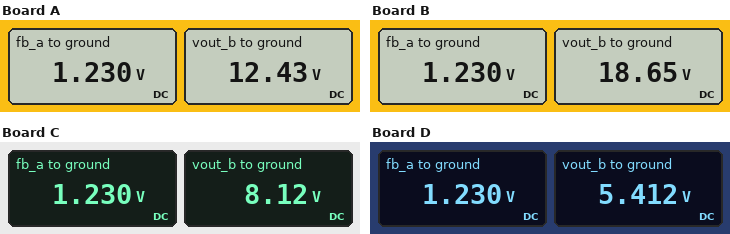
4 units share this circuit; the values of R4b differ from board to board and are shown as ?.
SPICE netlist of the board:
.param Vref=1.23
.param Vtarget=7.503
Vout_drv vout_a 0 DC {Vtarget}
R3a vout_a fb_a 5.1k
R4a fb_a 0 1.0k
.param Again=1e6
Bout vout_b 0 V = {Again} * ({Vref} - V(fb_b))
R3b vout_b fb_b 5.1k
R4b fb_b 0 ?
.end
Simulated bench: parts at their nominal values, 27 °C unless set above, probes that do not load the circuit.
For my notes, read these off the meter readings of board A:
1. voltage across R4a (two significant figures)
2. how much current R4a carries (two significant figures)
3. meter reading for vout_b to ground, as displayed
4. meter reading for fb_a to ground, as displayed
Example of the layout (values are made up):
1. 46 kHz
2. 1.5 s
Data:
1. 1.2 V
2. 1.2 mA
3. 12.43 V
4. 1.230 V
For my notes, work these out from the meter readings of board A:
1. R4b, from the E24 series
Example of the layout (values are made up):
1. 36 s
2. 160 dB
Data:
1. 560 Ω
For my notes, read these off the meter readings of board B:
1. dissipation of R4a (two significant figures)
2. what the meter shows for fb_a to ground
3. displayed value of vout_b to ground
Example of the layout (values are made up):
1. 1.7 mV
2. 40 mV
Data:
1. 1.5 mW
2. 1.230 V
3. 18.65 V
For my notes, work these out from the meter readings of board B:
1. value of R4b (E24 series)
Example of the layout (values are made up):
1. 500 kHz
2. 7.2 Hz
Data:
1. 360 Ω
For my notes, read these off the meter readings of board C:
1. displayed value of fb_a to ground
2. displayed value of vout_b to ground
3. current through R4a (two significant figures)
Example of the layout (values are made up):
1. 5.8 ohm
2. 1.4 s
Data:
1. 1.230 V
2. 8.12 V
3. 1.2 mA
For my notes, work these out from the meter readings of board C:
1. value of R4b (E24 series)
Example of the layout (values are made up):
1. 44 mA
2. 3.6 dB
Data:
1. 910 Ω
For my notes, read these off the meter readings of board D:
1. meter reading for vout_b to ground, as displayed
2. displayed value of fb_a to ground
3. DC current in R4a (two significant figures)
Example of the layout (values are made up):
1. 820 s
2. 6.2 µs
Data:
1. 5.412 V
2. 1.230 V
3. 1.2 mA
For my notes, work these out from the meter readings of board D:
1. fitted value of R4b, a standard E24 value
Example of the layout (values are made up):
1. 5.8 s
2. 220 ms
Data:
1. 1.5 kΩ
